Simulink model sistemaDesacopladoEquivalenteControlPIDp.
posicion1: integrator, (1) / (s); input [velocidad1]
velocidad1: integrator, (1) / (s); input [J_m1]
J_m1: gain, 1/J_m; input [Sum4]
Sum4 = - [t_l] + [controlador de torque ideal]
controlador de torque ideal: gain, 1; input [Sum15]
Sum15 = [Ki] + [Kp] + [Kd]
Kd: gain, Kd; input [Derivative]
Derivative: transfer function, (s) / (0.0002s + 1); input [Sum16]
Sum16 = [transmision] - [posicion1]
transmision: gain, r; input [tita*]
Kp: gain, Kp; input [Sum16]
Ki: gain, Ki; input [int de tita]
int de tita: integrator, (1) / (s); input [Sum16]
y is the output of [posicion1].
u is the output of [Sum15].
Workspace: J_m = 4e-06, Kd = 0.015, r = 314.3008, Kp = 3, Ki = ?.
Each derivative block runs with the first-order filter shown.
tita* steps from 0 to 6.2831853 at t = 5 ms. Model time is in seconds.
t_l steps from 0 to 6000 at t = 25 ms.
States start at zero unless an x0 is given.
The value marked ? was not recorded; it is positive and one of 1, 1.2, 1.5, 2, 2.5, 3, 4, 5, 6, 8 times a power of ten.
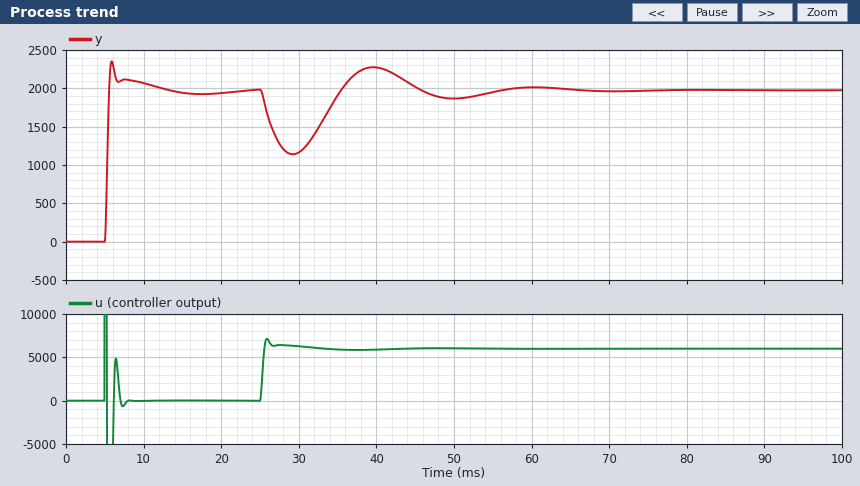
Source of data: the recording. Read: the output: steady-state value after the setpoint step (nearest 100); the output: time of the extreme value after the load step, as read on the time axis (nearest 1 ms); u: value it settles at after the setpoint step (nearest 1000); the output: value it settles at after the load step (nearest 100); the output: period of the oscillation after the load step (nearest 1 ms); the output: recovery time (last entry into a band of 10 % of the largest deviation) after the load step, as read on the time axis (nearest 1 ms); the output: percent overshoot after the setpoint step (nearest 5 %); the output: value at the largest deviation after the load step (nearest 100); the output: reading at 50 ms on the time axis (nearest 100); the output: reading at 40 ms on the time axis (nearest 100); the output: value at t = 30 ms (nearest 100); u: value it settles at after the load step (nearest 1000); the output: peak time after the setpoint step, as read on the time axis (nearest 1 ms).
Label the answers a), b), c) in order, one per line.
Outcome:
a) 2000
b) 29 ms
c) 0
d) 2000
e) 21 ms
f) 52 ms
g) 20 %
h) 1100
i) 1900
j) 2300
k) 1200
l) 6000
m) 6 ms
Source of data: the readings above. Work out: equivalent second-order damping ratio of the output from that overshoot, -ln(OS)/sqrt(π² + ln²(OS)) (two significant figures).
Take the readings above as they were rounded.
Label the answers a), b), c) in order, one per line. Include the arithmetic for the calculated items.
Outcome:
a) ln(0.2) = -1.609; 1.609 / sqrt(9.870 + 2.590) = 0.46
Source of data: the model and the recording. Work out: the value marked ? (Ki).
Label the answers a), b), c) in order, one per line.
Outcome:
a) 1500
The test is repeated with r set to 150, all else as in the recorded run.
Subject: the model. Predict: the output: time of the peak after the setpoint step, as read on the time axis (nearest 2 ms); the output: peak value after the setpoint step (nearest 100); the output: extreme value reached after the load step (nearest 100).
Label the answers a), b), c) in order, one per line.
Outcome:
a) 6 ms
b) 1100
c) 100
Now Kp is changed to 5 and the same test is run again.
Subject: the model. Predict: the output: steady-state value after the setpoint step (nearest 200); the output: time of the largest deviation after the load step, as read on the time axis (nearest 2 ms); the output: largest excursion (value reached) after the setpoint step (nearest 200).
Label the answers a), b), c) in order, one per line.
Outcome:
a) 2000
b) 28 ms
c) 2400
